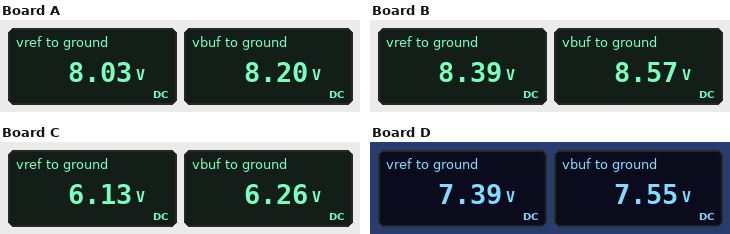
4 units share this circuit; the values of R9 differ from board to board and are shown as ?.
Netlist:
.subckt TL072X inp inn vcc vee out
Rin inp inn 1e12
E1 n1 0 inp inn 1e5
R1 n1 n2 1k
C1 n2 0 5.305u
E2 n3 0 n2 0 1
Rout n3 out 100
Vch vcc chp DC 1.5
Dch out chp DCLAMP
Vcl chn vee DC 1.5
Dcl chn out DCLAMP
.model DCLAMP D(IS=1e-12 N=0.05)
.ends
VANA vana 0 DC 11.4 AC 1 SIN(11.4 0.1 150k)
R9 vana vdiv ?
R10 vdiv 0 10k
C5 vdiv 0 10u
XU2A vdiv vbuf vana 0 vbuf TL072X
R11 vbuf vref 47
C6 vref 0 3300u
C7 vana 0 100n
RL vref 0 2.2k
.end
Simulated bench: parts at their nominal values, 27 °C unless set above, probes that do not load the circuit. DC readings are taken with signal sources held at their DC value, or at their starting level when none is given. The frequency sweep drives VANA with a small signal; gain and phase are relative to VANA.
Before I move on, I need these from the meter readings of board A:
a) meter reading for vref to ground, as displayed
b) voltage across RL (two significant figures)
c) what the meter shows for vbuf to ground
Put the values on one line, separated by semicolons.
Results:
8.03 V; 8.0 V; 8.20 V
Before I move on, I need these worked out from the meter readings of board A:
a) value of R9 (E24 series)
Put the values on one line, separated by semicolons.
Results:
3.9 kΩ
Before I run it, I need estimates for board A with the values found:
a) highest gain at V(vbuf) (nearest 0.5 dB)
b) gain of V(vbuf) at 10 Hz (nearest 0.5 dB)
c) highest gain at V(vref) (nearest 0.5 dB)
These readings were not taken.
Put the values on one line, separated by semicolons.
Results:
-3.0 dB; -9.0 dB; -3.0 dB
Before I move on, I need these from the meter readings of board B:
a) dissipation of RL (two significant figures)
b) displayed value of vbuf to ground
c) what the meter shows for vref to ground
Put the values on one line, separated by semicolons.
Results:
32 mW; 8.57 V; 8.39 V
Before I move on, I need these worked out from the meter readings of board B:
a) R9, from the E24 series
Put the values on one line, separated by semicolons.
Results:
3.3 kΩ
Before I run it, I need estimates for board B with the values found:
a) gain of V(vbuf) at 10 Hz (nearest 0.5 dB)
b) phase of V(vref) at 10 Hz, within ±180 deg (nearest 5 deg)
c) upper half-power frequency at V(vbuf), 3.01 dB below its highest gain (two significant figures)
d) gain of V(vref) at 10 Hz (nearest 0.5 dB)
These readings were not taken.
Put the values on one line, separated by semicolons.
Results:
-8.0 dB; -140 deg; 6.4 Hz; -27.5 dB
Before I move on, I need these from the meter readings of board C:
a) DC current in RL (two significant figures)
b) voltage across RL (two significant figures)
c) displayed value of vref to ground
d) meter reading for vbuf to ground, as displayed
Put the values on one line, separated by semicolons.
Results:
2.8 mA; 6.1 V; 6.13 V; 6.26 V
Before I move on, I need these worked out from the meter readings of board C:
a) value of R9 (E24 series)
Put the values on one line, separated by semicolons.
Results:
8.2 kΩ
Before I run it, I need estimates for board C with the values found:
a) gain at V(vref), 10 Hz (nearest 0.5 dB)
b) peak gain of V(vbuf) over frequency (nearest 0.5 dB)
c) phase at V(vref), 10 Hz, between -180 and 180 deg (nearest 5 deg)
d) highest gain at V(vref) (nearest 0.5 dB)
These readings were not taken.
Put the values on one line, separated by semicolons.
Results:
-34.5 dB; -5.0 dB; -155 deg; -5.5 dB
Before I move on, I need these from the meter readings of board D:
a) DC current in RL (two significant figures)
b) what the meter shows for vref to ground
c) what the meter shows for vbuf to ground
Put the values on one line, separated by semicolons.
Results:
3.4 mA; 7.39 V; 7.55 V
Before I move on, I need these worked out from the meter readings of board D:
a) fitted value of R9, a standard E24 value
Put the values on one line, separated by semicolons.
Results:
5.1 kΩ
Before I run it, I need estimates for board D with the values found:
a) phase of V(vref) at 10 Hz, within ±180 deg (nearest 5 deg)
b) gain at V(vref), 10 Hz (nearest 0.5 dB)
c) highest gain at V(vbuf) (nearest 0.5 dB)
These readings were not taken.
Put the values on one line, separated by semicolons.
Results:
-150 deg; -31.0 dB; -3.5 dB
